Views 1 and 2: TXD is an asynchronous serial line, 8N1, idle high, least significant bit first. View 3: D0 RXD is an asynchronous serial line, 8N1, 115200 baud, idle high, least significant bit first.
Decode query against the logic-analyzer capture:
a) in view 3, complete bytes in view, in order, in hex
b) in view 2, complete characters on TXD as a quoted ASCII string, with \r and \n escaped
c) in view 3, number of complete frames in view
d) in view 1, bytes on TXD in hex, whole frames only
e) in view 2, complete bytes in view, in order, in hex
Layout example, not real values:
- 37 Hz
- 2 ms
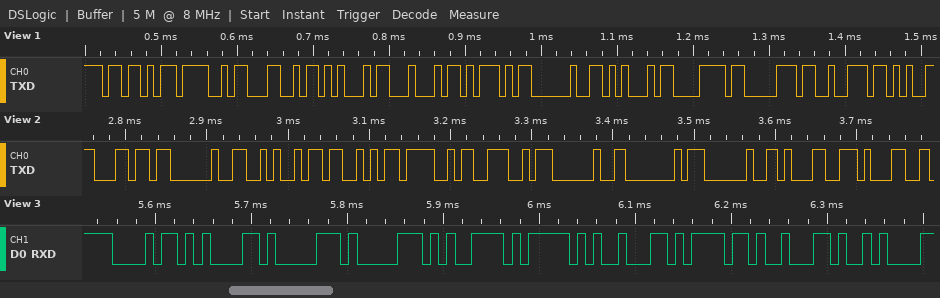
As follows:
- 68 61 70 70 79 5F 62 6F 62 0A
- "l JSON @ 11"
- 10
- 5B 4F 4C 45 44 5D 20 45 78 70 72
- 0x6C 0x20 0x4A 0x53 0x4F 0x4E 0x20 0x40 0x20 0x31 0x31
